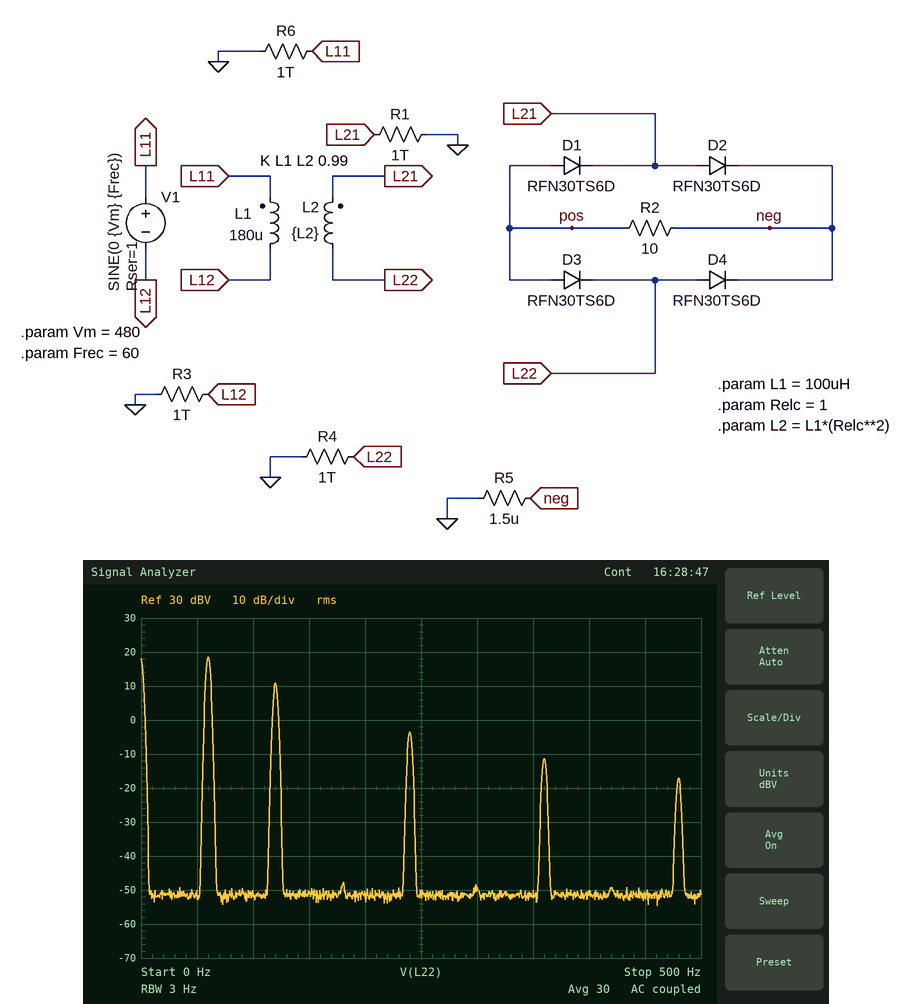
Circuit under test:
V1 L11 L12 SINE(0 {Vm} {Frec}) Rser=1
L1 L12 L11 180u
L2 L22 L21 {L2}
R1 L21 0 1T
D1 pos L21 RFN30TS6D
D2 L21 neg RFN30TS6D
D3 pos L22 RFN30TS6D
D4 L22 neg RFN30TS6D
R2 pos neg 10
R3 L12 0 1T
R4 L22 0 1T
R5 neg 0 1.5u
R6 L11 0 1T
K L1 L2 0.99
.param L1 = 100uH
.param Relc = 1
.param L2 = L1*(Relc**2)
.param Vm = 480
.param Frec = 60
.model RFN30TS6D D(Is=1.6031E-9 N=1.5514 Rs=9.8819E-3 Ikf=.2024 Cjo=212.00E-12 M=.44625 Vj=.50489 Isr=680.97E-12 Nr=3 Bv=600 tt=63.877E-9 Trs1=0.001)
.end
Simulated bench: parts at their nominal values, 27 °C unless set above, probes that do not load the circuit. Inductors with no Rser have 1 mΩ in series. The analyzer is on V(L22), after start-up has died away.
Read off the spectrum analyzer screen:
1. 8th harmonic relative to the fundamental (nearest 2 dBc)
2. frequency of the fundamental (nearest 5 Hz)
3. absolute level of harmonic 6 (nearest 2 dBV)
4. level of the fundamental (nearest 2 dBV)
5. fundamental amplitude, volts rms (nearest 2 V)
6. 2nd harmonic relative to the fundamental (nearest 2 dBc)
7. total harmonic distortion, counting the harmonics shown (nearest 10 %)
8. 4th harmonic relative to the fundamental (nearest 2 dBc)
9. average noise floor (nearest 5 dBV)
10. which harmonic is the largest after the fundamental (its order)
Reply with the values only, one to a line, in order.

-36 dBc
60 Hz
-12 dBV
18 dBV
8 V
-8 dBc
40 %
-22 dBc
-50 dBV
2
